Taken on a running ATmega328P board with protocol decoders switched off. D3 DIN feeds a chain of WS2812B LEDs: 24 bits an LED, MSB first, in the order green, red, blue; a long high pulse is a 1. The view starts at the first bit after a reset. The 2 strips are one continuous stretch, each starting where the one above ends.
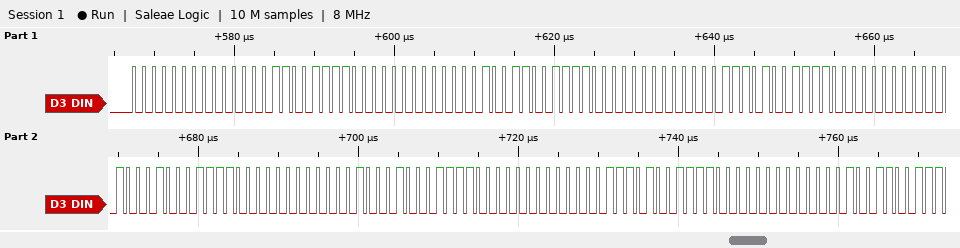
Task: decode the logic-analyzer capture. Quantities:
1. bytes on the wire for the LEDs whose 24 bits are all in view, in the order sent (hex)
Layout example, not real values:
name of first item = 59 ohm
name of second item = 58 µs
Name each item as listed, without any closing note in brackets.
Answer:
bytes on the wire for the LEDs whose 24 bits are all in view, in the order sent = 00 03 3C 00 13 3C 00 1D 3C 00 22 3C 00 22 3C 00 1D 3C
